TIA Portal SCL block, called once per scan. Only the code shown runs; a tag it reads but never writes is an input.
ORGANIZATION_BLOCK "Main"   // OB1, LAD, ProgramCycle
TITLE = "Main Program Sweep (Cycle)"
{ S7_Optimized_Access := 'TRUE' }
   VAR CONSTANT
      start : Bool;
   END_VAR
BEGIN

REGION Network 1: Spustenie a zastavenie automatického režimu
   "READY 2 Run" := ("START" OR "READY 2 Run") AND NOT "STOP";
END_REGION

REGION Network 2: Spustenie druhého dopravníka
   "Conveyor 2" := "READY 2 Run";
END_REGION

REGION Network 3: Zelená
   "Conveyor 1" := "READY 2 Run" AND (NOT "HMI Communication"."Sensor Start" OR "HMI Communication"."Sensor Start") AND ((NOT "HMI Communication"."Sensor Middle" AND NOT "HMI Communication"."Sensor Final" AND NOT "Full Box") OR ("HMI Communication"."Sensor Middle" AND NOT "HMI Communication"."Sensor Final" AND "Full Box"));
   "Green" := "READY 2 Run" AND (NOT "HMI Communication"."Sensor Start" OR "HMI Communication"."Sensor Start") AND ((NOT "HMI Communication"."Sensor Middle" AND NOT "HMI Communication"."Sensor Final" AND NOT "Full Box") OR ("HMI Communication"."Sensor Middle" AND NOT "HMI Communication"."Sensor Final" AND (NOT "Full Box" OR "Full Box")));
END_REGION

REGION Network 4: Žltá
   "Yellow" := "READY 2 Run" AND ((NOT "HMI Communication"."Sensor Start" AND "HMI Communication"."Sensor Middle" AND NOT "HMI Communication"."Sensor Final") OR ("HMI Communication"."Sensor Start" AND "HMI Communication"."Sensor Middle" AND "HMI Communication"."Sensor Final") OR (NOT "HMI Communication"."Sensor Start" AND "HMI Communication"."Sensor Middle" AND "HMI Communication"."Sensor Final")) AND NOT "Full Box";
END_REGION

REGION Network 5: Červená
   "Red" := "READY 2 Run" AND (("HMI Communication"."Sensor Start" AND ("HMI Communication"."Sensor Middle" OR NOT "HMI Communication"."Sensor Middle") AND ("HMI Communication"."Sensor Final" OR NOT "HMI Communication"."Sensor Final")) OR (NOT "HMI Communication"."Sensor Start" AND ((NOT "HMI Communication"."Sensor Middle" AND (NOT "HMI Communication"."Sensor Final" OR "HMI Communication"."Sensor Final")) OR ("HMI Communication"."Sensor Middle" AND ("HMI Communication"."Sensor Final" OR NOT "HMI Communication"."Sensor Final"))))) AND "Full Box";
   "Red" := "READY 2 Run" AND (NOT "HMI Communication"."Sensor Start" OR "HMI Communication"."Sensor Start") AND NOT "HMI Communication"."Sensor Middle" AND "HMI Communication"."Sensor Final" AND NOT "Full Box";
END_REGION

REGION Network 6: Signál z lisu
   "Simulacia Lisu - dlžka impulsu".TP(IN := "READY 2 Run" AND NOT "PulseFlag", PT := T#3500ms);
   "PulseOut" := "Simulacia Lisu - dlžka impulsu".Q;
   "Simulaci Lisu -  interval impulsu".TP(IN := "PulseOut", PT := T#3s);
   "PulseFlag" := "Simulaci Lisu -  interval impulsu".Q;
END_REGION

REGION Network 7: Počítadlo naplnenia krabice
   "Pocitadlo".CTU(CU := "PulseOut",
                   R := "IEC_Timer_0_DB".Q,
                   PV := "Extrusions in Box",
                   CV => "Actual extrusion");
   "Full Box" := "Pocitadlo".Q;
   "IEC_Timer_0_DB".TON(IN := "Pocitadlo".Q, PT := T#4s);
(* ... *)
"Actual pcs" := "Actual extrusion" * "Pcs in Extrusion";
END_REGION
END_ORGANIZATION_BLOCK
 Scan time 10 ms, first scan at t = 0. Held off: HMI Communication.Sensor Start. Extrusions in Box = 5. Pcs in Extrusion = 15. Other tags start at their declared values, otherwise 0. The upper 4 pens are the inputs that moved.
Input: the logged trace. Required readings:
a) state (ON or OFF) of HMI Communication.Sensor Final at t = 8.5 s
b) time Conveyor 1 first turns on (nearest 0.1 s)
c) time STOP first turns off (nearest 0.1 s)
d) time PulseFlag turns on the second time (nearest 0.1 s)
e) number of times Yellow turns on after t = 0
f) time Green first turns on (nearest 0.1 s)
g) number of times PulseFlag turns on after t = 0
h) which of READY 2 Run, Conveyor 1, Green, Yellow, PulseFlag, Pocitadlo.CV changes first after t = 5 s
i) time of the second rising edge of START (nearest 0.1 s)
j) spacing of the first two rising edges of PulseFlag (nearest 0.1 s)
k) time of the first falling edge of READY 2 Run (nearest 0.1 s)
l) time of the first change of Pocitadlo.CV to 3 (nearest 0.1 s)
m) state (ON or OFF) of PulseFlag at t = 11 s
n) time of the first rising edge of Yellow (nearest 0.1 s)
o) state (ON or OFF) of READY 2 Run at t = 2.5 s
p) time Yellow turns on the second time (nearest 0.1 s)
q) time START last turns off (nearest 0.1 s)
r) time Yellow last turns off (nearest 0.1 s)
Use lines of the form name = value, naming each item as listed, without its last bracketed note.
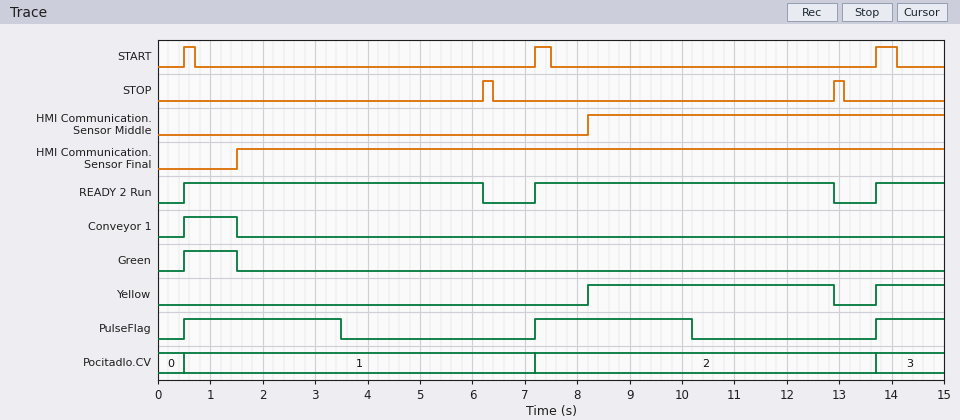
state (ON or OFF) of HMI Communication.Sensor Final at t = 8.5 s = ON
time Conveyor 1 first turns on = 0.5 s
time STOP first turns off = 6.4 s
time PulseFlag turns on the second time = 7.2 s
number of times Yellow turns on after t = 0 = 2
time Green first turns on = 0.5 s
number of times PulseFlag turns on after t = 0 = 3
which of READY 2 Run, Conveyor 1, Green, Yellow, PulseFlag, Pocitadlo.CV changes first after t = 5 s = READY 2 Run
time of the second rising edge of START = 7.2 s
spacing of the first two rising edges of PulseFlag = 6.7 s
time of the first falling edge of READY 2 Run = 6.2 s
time of the first change of Pocitadlo.CV to 3 = 13.7 s
state (ON or OFF) of PulseFlag at t = 11 s = OFF
time of the first rising edge of Yellow = 8.2 s
state (ON or OFF) of READY 2 Run at t = 2.5 s = ON
time Yellow turns on the second time = 13.7 s
time START last turns off = 14.1 s
time Yellow last turns off = 12.9 s
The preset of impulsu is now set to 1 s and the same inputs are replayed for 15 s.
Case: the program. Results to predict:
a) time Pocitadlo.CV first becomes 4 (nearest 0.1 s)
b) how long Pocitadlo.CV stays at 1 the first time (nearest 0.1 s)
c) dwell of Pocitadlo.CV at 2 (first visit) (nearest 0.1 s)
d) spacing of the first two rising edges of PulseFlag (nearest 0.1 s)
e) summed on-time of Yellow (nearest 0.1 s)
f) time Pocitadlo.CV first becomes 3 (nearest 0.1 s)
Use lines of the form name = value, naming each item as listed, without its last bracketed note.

time Pocitadlo.CV first becomes 4 = 10.2 s
how long Pocitadlo.CV stays at 1 the first time = 3.0 s
dwell of Pocitadlo.CV at 2 (first visit) = 3.7 s
spacing of the first two rising edges of PulseFlag = 3.0 s
summed on-time of Yellow = 4.7 s
time Pocitadlo.CV first becomes 3 = 7.2 s
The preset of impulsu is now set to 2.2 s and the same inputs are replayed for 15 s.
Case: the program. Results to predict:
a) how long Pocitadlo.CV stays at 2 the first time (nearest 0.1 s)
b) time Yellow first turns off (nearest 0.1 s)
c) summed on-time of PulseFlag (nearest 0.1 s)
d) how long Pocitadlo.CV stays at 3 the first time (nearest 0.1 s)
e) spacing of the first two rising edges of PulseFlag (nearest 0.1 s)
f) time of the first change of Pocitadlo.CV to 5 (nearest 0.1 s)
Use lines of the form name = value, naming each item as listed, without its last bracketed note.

how long Pocitadlo.CV stays at 2 the first time = 3.7 s
time Yellow first turns off = 12.9 s
summed on-time of PulseFlag = 13.3 s
how long Pocitadlo.CV stays at 3 the first time = 3.0 s
spacing of the first two rising edges of PulseFlag = 3.0 s
time of the first change of Pocitadlo.CV to 5 = 13.7 s
